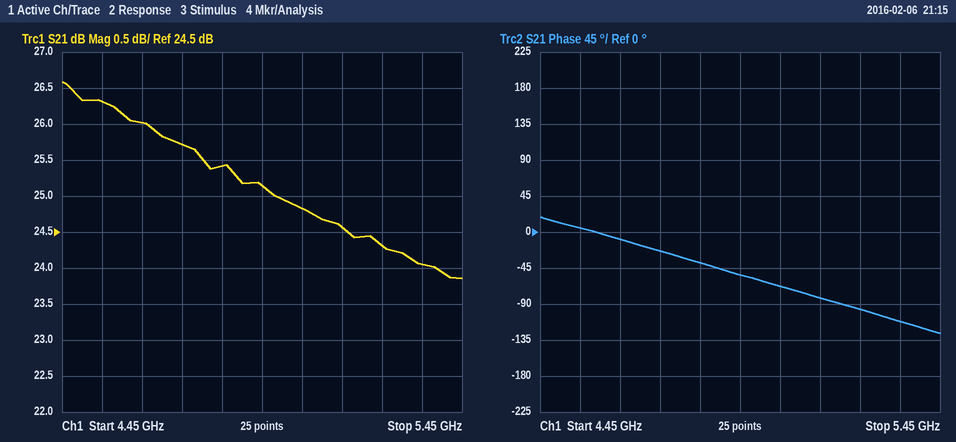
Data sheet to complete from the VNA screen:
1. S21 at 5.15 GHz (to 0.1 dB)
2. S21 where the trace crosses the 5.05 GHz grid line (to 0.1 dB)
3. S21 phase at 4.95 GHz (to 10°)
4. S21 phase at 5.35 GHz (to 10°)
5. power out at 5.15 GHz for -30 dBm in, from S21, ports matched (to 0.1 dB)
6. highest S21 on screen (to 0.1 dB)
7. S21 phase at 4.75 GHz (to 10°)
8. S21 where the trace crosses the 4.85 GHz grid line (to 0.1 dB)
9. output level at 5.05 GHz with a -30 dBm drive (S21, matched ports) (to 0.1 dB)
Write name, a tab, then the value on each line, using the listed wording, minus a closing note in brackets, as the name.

S21 at 5.15 GHz	24.6 dB
S21 where the trace crosses the 5.05 GHz grid line	24.8 dB
S21 phase at 4.95 GHz	-50°
S21 phase at 5.35 GHz	-110°
power out at 5.15 GHz for -30 dBm in, from S21, ports matched	-5.4 dBm
highest S21 on screen	26.6 dB
S21 phase at 4.75 GHz	-20°
S21 where the trace crosses the 4.85 GHz grid line	25.4 dB
output level at 5.05 GHz with a -30 dBm drive (S21, matched ports)	-5.2 dBm
